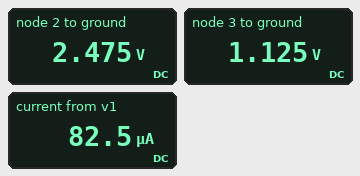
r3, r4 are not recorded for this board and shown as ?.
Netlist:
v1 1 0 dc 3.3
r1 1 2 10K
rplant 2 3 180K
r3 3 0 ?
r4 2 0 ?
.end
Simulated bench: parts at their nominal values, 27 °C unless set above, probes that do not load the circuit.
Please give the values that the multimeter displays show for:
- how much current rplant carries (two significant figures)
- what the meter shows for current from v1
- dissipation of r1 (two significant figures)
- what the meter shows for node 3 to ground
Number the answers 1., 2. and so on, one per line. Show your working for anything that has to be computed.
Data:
1. (2.475 V - 1.125 V) / 180 kΩ = 7.5 µA
2. 82.5 µA
3. (3.3 V - 2.475 V)^2 / 10 kΩ = 68 µW
4. 1.125 V
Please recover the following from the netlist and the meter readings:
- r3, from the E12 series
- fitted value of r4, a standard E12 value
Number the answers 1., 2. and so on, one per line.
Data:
1. 150 kΩ
2. 33 kΩ
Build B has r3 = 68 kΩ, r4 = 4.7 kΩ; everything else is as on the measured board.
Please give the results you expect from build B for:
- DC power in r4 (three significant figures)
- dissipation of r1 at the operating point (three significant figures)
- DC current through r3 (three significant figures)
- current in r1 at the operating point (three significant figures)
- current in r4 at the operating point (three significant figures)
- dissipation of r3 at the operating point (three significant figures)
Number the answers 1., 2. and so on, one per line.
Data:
1. 231 µW
2. 510 µW
3. 4.20 µA
4. 226 µA
5. 222 µA
6. 1.20 µW
